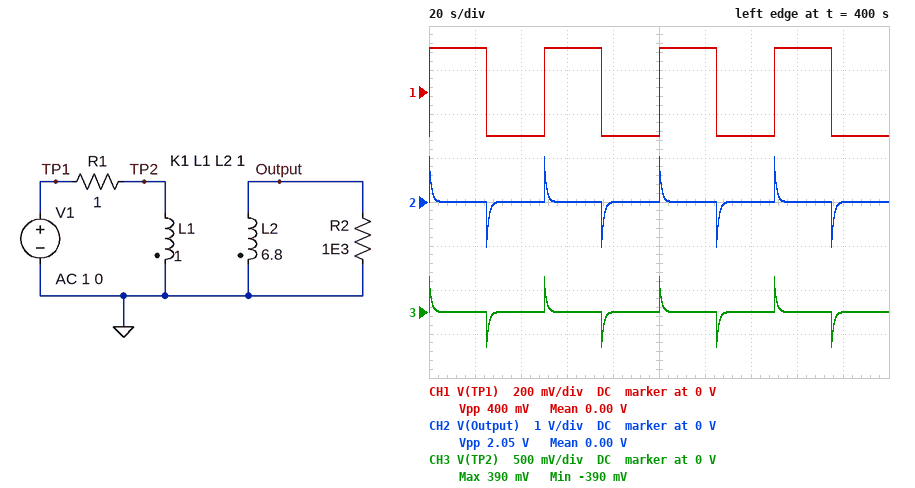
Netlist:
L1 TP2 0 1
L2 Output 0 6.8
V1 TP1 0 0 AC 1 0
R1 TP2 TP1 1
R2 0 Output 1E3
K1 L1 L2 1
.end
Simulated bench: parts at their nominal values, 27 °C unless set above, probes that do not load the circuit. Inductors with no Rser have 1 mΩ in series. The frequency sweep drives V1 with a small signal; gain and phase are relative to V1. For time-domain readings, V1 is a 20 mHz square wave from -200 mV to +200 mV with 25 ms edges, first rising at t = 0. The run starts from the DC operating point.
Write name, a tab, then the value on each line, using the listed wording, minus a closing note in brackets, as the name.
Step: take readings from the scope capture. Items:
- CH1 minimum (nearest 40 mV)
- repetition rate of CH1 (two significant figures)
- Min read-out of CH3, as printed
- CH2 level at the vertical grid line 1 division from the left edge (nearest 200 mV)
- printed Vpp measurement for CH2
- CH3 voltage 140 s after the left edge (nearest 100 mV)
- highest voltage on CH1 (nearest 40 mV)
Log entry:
CH1 minimum	-200 mV
repetition rate of CH1	20 mHz
Min read-out of CH3, as printed	-390 mV
CH2 level at the vertical grid line 1 division from the left edge	0 V
printed Vpp measurement for CH2	2.05 V
CH3 voltage 140 s after the left edge	0 V
highest voltage on CH1	200 mV
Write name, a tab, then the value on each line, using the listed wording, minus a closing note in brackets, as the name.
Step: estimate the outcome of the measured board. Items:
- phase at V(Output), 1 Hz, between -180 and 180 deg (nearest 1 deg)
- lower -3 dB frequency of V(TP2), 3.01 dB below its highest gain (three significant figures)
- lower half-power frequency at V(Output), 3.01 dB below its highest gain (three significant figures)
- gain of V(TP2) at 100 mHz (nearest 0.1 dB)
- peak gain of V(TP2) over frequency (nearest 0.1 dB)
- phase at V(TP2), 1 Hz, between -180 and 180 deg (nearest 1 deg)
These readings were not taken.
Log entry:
phase at V(Output), 1 Hz, between -180 and 180 deg	9 deg
lower -3 dB frequency of V(TP2), 3.01 dB below its highest gain	158 mHz
lower half-power frequency at V(Output), 3.01 dB below its highest gain	158 mHz
gain of V(TP2) at 100 mHz	-5.5 dB
peak gain of V(TP2) over frequency	-0.1 dB
phase at V(TP2), 1 Hz, between -180 and 180 deg	9 deg
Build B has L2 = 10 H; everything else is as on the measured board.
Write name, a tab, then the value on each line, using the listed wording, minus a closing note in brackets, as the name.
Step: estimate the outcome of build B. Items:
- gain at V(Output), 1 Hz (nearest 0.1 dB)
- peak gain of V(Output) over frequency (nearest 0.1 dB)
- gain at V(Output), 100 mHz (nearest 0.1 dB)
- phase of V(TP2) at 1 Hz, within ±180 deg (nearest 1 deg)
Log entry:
gain at V(Output), 1 Hz	9.8 dB
peak gain of V(Output) over frequency	9.9 dB
gain at V(Output), 100 mHz	4.5 dB
phase of V(TP2) at 1 Hz, within ±180 deg	9 deg
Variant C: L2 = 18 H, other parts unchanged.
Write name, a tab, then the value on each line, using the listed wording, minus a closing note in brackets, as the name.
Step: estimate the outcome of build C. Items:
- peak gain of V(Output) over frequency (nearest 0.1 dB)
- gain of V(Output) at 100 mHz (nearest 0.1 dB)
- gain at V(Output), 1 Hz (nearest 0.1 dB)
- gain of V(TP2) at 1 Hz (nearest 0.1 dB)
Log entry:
peak gain of V(Output) over frequency	12.4 dB
gain of V(Output) at 100 mHz	7.0 dB
gain at V(Output), 1 Hz	12.3 dB
gain of V(TP2) at 1 Hz	-0.3 dB
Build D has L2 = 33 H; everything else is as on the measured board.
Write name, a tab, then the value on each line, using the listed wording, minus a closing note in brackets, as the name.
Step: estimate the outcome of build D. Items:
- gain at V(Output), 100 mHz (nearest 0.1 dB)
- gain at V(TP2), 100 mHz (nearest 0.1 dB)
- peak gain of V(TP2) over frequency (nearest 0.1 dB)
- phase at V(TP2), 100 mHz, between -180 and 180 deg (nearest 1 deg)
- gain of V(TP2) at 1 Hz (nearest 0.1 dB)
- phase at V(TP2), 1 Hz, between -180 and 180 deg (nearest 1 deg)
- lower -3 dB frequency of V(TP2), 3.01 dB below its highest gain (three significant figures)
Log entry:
gain at V(Output), 100 mHz	9.6 dB
gain at V(TP2), 100 mHz	-5.6 dB
peak gain of V(TP2) over frequency	-0.3 dB
phase at V(TP2), 100 mHz, between -180 and 180 deg	57 deg
gain of V(TP2) at 1 Hz	-0.4 dB
phase at V(TP2), 1 Hz, between -180 and 180 deg	9 deg
lower -3 dB frequency of V(TP2), 3.01 dB below its highest gain	154 mHz
